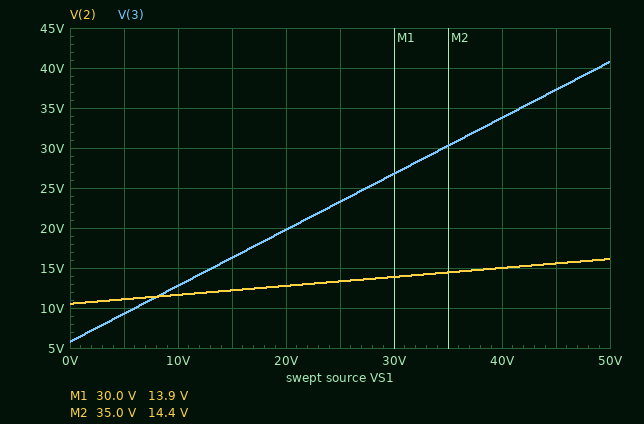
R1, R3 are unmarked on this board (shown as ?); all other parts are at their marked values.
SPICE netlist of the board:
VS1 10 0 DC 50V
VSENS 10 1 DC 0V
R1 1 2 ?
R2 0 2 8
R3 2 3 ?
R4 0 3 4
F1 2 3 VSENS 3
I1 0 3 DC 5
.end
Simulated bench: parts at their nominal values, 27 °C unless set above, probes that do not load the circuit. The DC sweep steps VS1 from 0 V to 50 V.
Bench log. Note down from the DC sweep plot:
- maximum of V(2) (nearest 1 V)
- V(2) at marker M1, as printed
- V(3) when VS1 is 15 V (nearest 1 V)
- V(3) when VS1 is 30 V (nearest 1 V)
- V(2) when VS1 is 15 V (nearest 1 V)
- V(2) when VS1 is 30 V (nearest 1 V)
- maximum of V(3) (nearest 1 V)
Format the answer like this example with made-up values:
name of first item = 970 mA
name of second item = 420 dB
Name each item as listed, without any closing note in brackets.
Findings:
maximum of V(2) = 16 V
V(2) at marker M1, as printed = 13.9 V
V(3) when VS1 is 15 V = 16 V
V(3) when VS1 is 30 V = 27 V
V(2) when VS1 is 15 V = 12 V
V(2) when VS1 is 30 V = 14 V
maximum of V(3) = 41 V
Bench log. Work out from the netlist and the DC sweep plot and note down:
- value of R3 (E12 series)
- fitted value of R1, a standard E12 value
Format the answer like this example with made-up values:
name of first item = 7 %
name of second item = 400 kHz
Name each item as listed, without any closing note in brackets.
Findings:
value of R3 = 1.5 Ω
fitted value of R1, a standard E12 value = 4.7 Ω
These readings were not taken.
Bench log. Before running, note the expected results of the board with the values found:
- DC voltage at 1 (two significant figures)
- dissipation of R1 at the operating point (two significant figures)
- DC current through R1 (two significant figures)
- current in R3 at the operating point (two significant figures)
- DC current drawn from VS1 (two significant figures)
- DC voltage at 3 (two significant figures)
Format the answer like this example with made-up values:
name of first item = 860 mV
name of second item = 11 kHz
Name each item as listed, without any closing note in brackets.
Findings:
DC voltage at 1 = 50 V
dissipation of R1 at the operating point = 240 W
DC current through R1 = 7.2 A
current in R3 at the operating point = 16 A
DC current drawn from VS1 = 7.2 A
DC voltage at 3 = 41 V
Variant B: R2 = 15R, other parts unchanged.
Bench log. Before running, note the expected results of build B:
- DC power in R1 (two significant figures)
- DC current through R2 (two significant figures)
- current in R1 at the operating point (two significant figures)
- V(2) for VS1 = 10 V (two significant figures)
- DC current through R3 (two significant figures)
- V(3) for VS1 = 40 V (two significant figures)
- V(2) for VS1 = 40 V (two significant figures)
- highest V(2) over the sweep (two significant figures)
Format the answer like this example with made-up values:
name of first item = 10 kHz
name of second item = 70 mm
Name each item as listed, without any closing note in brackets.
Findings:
DC power in R1 = 200 W
DC current through R2 = 1.3 A
current in R1 at the operating point = 6.5 A
V(2) for VS1 = 10 V = 14 V
DC current through R3 = 14 A
V(3) for VS1 = 40 V = 34 V
V(2) for VS1 = 40 V = 18 V
highest V(2) over the sweep = 19 V
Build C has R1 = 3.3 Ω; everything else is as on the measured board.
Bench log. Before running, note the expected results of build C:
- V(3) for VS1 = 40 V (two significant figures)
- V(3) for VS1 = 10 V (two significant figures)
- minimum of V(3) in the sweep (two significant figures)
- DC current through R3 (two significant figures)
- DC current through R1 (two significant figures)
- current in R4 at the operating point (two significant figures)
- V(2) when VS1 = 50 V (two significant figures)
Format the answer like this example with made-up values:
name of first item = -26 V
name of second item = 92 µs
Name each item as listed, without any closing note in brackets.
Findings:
V(3) for VS1 = 40 V = 41 V
V(3) for VS1 = 10 V = 12 V
minimum of V(3) in the sweep = 2.8 V
DC current through R3 = 22 A
DC current through R1 = 9.8 A
current in R4 at the operating point = 13 A
V(2) when VS1 = 50 V = 18 V
